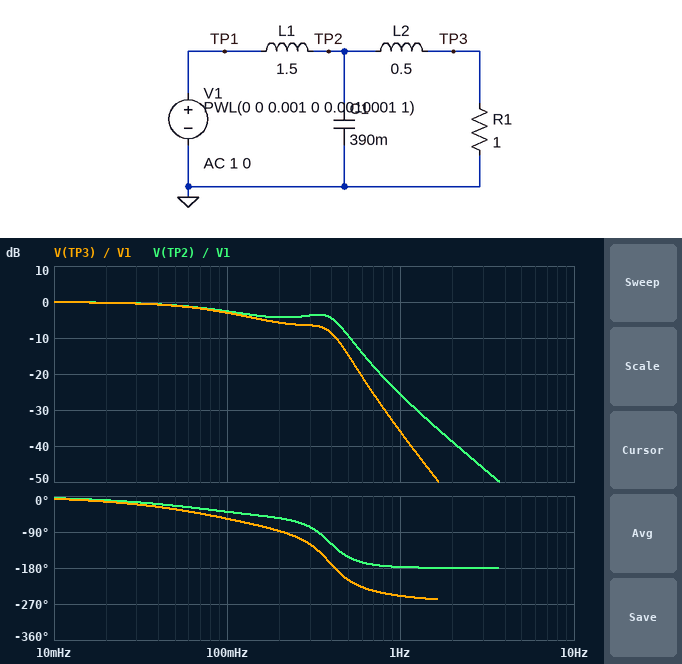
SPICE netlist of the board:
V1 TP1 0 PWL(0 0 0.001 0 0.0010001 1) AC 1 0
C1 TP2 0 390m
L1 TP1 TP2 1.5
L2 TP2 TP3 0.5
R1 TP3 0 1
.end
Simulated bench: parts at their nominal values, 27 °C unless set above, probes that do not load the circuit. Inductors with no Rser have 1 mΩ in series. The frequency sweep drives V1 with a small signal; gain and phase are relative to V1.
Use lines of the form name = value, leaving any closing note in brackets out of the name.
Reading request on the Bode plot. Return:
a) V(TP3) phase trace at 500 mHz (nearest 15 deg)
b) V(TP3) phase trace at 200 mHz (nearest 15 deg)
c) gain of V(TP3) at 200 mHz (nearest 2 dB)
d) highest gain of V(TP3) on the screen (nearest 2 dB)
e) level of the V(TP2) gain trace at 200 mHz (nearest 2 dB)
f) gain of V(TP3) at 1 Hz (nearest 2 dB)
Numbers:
V(TP3) phase trace at 500 mHz = -210 deg
V(TP3) phase trace at 200 mHz = -90 deg
gain of V(TP3) at 200 mHz = -6 dB
highest gain of V(TP3) on the screen = 0 dB
level of the V(TP2) gain trace at 200 mHz = -4 dB
gain of V(TP3) at 1 Hz = -36 dB
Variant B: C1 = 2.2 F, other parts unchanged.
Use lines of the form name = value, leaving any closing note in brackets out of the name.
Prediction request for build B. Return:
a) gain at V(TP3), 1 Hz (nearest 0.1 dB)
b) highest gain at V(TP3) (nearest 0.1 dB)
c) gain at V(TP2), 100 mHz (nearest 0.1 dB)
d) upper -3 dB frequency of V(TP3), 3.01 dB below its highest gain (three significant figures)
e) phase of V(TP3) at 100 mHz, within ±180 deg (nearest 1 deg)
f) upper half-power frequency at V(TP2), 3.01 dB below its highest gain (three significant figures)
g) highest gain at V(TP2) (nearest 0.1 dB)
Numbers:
gain at V(TP3), 1 Hz = -52.4 dB
highest gain at V(TP3) = 1.8 dB
gain at V(TP2), 100 mHz = 1.3 dB
upper -3 dB frequency of V(TP3), 3.01 dB below its highest gain = 118 mHz
phase of V(TP3) at 100 mHz, within ±180 deg = -110 deg
upper half-power frequency at V(TP2), 3.01 dB below its highest gain = 120 mHz
highest gain at V(TP2) = 2.1 dB
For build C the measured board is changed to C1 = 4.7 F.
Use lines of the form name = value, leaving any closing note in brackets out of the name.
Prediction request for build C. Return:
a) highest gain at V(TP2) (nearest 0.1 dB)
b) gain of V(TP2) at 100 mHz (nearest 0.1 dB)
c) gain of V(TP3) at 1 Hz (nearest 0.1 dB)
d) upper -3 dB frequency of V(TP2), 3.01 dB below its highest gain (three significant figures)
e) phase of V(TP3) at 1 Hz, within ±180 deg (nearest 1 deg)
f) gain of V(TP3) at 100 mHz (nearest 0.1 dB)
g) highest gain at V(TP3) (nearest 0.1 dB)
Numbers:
highest gain at V(TP2) = 5.1 dB
gain of V(TP2) at 100 mHz = -4.8 dB
gain of V(TP3) at 1 Hz = -59.1 dB
upper -3 dB frequency of V(TP2), 3.01 dB below its highest gain = 74.9 mHz
phase of V(TP3) at 1 Hz, within ±180 deg = 108 deg
gain of V(TP3) at 100 mHz = -5.2 dB
highest gain at V(TP3) = 5.0 dB
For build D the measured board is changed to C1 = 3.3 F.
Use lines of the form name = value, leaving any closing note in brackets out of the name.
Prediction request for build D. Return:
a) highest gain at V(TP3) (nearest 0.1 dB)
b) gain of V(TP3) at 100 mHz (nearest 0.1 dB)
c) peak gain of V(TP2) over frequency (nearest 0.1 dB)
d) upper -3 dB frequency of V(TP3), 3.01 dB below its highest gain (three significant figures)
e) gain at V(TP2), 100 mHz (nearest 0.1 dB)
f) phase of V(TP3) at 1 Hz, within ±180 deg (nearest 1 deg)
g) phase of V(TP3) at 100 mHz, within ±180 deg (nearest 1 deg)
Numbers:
highest gain at V(TP3) = 3.5 dB
gain of V(TP3) at 100 mHz = -1.2 dB
peak gain of V(TP2) over frequency = 3.7 dB
upper -3 dB frequency of V(TP3), 3.01 dB below its highest gain = 92.2 mHz
gain at V(TP2), 100 mHz = -0.8 dB
phase of V(TP3) at 1 Hz, within ±180 deg = 108 deg
phase of V(TP3) at 100 mHz, within ±180 deg = -146 deg
